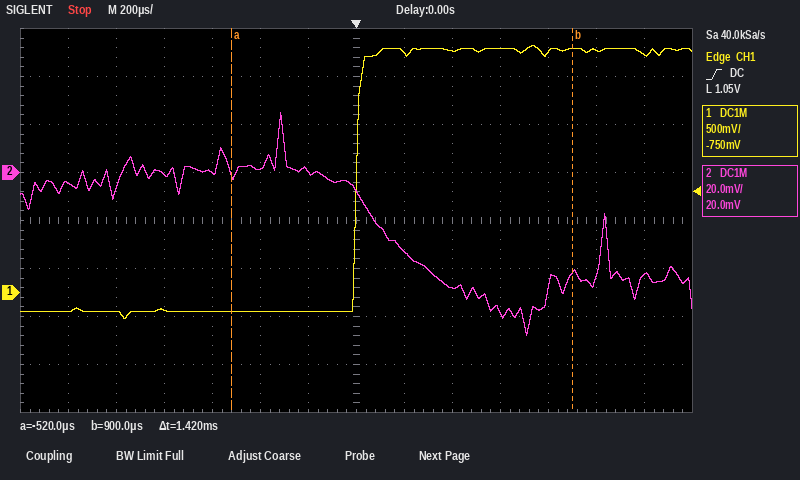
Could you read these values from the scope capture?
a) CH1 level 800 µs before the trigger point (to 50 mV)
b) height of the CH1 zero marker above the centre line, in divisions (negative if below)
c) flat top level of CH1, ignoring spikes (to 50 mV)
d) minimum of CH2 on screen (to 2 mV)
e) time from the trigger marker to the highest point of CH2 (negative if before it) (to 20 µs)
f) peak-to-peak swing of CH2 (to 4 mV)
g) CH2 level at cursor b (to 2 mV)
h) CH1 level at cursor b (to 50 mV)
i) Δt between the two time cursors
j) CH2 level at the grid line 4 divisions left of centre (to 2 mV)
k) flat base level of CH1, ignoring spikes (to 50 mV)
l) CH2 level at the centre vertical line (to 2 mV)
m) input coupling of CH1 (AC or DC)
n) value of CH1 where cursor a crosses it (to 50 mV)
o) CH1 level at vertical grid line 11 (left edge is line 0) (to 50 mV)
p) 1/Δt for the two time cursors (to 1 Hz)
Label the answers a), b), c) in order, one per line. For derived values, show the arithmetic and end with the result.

a) -200 mV
b) -1.5 div
c) 2.55 V
d) -68 mV
e) -320 µs
f) 92 mV
g) -42 mV
h) 2.55 V
i) 1.42 ms
j) 0 mV
k) -200 mV
l) -8 mV
m) DC
n) -200 mV
o) 2.50 V
p) 1 / 1.42 ms ≈ 704 Hz
